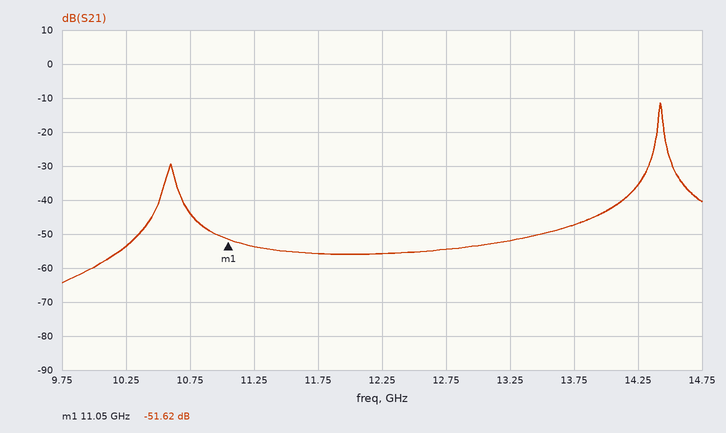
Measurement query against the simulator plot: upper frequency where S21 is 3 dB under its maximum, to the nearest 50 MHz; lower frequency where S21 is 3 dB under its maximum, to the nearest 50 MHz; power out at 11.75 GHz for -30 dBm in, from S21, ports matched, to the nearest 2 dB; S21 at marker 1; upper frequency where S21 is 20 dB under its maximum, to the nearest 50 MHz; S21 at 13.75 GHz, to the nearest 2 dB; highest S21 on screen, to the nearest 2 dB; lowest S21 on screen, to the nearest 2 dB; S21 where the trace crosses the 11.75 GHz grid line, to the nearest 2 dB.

14.45 GHz
14.40 GHz
-86 dBm
-51.62 dB
14.55 GHz
-48 dB
-12 dB
-64 dB
-56 dB
